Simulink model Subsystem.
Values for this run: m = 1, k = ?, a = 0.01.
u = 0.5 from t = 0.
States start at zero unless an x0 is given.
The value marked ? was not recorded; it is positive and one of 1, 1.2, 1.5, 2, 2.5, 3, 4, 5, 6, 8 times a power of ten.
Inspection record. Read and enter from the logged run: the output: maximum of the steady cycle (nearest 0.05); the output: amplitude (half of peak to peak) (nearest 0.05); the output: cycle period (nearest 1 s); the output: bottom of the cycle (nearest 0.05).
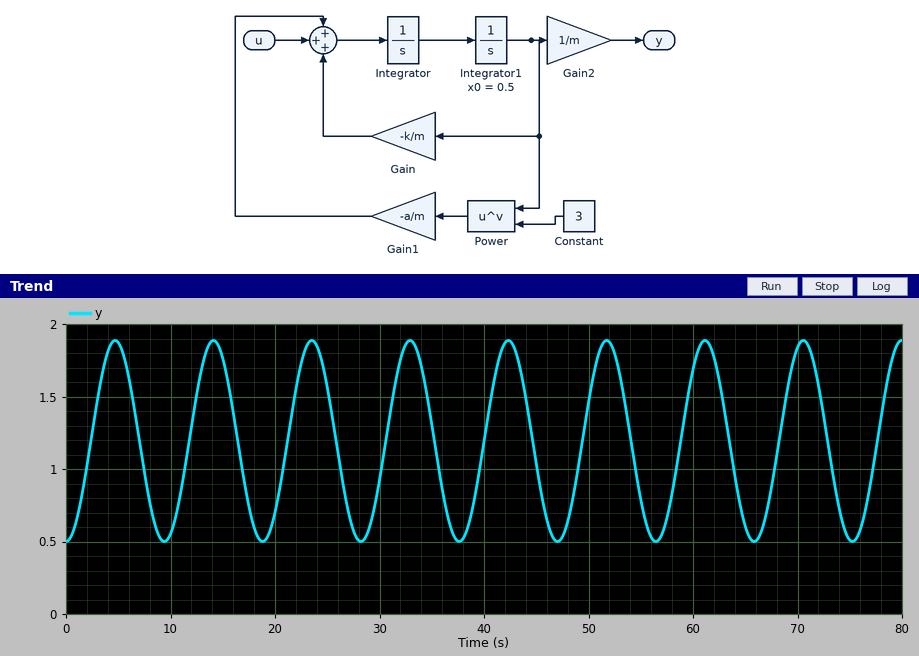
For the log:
1.90
0.70
9 s
0.50
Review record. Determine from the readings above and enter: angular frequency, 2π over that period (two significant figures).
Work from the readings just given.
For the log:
0.70 rad/s
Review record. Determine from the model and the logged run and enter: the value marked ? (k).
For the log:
0.4
